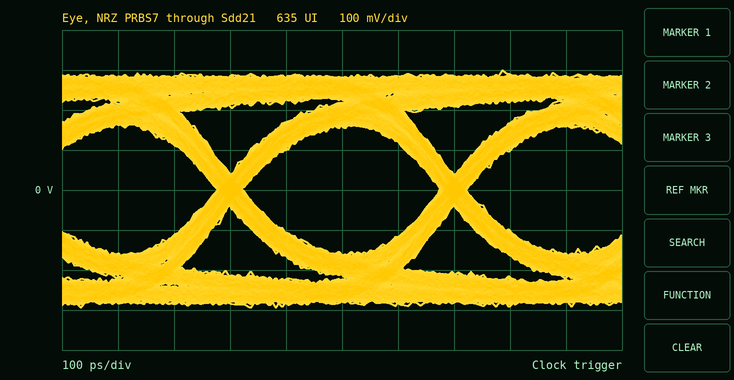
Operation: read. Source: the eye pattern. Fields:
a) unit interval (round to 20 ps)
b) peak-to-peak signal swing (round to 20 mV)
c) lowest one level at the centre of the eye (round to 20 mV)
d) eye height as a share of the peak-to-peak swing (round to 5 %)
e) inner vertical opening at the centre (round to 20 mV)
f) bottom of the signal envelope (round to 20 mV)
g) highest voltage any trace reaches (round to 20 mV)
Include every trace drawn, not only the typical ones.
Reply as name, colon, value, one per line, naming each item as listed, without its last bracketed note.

unit interval: 400 ps
peak-to-peak signal swing: 600 mV
lowest one level at the centre of the eye: 160 mV
eye height as a share of the peak-to-peak swing: 55 %
inner vertical opening at the centre: 320 mV
bottom of the signal envelope: -300 mV
highest voltage any trace reaches: 300 mV
